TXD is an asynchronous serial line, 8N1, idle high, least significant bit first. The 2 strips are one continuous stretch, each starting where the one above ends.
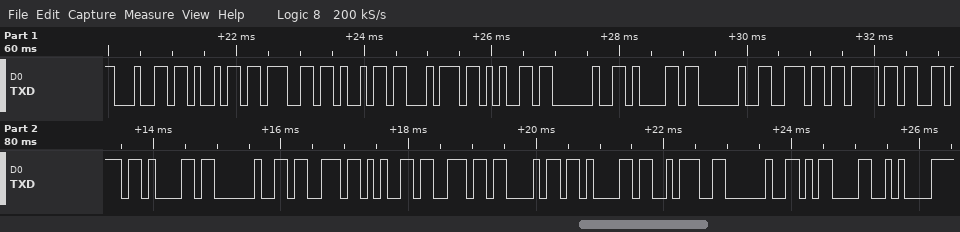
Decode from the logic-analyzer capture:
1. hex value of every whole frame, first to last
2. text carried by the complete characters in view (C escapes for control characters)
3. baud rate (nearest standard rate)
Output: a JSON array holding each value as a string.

["0x64 0x69 0x67 0x69 0x74 0x65 0x20 0x61 0x20 0x6E 0x6F 0x76 0x61 0x20 0x73 0x65 0x6E 0x68 0x61 0x3A 0x20 0x0D 0x0A", "\"digite a nova senha: \\r\\n\"", "9600 baud"]
